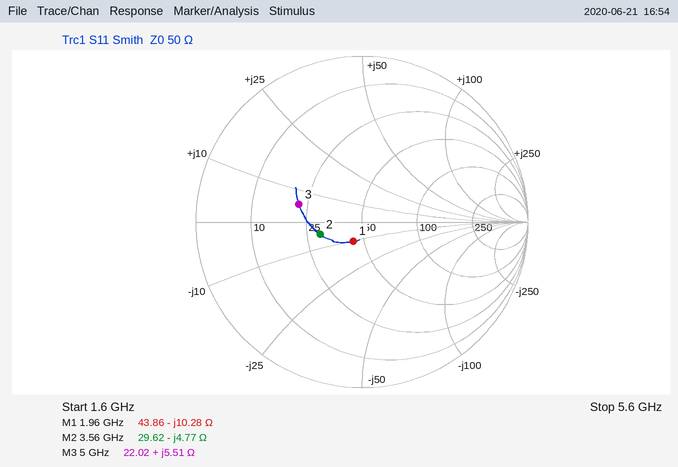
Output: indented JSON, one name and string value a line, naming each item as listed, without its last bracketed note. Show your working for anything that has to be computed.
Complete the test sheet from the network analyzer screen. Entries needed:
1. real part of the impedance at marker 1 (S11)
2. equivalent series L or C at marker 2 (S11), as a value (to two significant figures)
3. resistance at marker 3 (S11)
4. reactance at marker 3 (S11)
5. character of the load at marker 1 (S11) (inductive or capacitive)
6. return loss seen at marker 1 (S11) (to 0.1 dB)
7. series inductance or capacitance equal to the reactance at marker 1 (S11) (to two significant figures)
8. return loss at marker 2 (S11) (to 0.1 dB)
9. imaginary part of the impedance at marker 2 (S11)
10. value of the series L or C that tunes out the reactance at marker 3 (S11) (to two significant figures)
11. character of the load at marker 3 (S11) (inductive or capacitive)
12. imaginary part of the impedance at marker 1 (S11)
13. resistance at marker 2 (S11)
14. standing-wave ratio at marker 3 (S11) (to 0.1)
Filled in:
{
  "real part of the impedance at marker 1": "43.86 Ω",
  "equivalent series L or C at marker 2 (S11), as a value": "C = 1/(2π × 3.56 GHz × 4.77 Ω) ≈ 9.4 pF",
  "resistance at marker 3": "22.02 Ω",
  "reactance at marker 3": "+5.51 Ω",
  "character of the load at marker 1 (S11)": "capacitive",
  "return loss seen at marker 1 (S11)": "17.9 dB",
  "series inductance or capacitance equal to the reactance at marker 1 (S11)": "C = 1/(2π × 1.96 GHz × 10.28 Ω) ≈ 7.9 pF",
  "return loss at marker 2 (S11)": "11.6 dB",
  "imaginary part of the impedance at marker 2": "-4.77 Ω",
  "value of the series L or C that tunes out the reactance at marker 3 (S11)": "C = 1/(2π × 5 GHz × 5.51 Ω) ≈ 5.8 pF",
  "character of the load at marker 3 (S11)": "inductive",
  "imaginary part of the impedance at marker 1": "-10.28 Ω",
  "resistance at marker 2": "29.62 Ω",
  "standing-wave ratio at marker 3 (S11)": "2.3"
}
